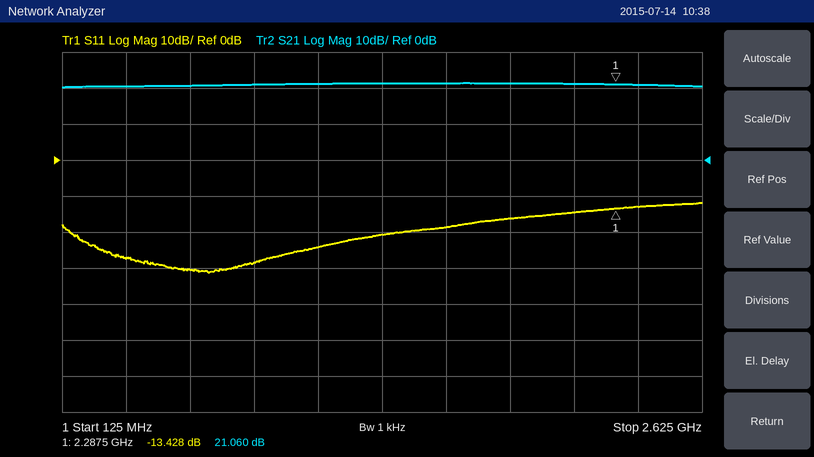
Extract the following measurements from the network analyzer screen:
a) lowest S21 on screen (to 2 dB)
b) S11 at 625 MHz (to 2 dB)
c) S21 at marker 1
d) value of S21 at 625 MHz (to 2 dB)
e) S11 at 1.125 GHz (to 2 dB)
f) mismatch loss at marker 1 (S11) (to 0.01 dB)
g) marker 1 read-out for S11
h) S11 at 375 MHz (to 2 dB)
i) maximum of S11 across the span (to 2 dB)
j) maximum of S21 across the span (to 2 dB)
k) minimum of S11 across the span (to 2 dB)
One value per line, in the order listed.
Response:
20 dB
-30 dB
21.060 dB
20 dB
-24 dB
0.20 dB
-13.428 dB
-28 dB
-12 dB
22 dB
-32 dB
